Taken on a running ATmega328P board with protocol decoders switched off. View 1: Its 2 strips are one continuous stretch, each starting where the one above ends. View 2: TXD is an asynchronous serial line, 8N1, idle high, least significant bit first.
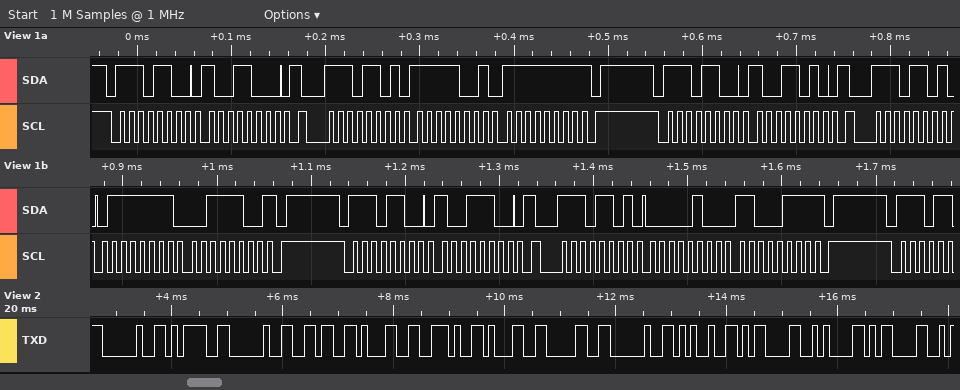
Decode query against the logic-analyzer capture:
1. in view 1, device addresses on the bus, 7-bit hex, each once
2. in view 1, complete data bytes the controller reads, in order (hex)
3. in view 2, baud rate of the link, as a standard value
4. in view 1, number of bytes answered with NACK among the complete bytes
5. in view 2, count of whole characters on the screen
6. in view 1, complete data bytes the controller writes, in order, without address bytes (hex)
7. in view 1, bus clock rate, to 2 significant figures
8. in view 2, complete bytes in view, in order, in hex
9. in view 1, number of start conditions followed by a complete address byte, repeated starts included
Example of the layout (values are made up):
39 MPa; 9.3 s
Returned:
0x76; F9 FF 7F 3C 04 C7; 9600 baud; 3; 13; 98 9A 9C; 100 kHz; 20 3D 20 36 31 2E 31 30 20 25 0D 0A 0D; 6
